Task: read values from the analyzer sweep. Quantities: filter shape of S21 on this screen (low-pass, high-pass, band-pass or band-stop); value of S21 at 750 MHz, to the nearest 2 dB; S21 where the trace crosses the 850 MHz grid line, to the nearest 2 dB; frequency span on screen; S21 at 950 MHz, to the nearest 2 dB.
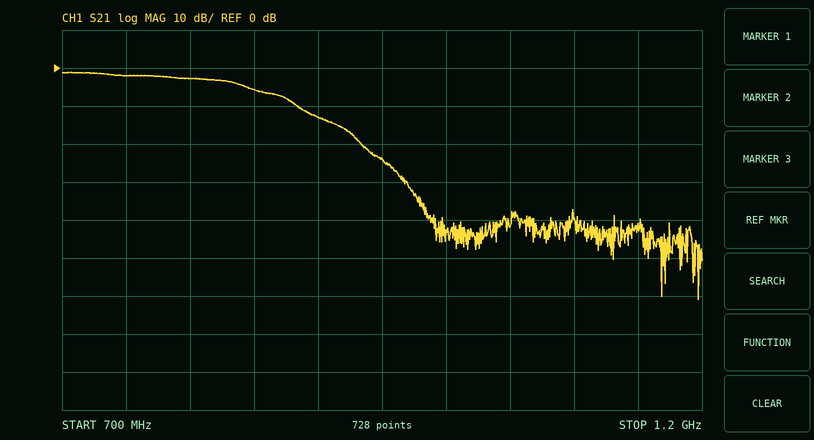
low-pass
-2 dB
-6 dB
500 MHz
-24 dB
